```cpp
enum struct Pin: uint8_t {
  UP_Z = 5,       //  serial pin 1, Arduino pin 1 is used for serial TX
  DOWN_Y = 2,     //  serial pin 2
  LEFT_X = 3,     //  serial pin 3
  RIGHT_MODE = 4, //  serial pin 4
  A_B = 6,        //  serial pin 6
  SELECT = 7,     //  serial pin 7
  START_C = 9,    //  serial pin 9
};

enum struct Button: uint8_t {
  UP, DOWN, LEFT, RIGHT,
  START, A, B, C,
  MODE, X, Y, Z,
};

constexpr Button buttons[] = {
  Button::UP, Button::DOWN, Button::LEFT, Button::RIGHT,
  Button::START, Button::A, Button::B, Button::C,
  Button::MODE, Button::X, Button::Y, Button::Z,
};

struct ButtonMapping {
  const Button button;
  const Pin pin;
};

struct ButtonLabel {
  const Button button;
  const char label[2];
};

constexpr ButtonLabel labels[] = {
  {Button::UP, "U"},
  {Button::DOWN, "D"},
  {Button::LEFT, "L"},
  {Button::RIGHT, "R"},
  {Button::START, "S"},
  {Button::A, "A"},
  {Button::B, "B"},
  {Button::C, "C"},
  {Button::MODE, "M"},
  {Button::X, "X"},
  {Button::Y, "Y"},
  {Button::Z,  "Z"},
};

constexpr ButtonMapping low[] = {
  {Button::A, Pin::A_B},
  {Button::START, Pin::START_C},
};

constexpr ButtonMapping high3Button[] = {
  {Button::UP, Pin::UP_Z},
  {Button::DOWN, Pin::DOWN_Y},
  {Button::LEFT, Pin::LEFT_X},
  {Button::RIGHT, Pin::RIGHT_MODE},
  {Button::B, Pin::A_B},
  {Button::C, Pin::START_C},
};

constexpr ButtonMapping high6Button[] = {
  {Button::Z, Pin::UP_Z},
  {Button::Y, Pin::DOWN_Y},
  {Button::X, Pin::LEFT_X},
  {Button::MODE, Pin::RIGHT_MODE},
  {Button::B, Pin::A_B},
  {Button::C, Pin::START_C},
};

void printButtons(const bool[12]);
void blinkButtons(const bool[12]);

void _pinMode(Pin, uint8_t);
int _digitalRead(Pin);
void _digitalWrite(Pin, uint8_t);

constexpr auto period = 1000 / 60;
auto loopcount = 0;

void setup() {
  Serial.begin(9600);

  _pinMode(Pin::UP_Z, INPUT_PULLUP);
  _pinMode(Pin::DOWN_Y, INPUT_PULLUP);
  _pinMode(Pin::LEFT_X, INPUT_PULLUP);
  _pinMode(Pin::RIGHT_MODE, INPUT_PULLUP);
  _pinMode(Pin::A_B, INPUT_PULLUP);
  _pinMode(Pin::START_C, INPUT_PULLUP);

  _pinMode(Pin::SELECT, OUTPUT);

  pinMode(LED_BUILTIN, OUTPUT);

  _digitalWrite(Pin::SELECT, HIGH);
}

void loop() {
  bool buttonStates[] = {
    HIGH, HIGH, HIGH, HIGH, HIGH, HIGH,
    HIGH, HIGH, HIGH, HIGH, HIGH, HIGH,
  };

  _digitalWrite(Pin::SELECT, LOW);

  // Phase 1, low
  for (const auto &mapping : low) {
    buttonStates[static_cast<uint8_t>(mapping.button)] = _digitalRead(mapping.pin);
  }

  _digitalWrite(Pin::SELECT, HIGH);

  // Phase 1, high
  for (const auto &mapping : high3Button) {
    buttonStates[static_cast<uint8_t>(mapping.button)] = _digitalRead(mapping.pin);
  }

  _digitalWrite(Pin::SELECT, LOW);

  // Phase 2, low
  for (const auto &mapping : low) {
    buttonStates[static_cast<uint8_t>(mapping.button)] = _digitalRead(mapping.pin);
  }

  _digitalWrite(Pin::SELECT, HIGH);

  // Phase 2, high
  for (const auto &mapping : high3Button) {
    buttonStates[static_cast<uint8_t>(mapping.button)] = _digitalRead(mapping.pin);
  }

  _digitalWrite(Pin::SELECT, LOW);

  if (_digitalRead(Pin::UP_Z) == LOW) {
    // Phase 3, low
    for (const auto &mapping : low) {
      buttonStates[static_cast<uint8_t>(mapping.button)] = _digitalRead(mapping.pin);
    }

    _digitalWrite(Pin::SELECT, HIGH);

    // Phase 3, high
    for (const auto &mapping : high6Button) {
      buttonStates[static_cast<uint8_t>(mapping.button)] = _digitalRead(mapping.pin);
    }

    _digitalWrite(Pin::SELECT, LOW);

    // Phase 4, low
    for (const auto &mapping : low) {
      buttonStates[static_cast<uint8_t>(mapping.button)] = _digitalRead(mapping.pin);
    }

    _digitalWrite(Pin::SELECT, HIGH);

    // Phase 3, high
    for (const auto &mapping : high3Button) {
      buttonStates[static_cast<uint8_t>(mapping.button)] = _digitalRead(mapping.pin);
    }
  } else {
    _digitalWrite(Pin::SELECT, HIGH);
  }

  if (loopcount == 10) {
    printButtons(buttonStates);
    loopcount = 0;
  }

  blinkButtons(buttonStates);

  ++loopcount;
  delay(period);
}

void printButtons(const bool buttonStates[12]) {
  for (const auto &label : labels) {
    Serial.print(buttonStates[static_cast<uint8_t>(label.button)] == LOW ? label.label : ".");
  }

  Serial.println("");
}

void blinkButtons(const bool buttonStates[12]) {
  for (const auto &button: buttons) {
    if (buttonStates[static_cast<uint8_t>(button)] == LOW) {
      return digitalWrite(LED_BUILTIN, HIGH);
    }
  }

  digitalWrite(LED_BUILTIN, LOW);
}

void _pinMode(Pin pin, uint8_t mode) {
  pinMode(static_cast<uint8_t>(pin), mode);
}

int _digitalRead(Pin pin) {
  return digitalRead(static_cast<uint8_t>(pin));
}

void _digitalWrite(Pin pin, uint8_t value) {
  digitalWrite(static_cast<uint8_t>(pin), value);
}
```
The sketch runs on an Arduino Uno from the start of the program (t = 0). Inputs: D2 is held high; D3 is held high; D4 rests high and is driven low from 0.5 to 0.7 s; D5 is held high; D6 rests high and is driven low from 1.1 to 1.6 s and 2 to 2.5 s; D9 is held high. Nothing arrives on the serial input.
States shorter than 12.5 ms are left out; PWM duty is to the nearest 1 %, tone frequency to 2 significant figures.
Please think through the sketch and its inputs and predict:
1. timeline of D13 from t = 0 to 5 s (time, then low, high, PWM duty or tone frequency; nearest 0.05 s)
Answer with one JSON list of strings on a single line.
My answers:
["0 s low; 0.5 s high; 0.7 s low; 1.1 s high; 1.6 s low; 2 s high; 2.5 s low"]
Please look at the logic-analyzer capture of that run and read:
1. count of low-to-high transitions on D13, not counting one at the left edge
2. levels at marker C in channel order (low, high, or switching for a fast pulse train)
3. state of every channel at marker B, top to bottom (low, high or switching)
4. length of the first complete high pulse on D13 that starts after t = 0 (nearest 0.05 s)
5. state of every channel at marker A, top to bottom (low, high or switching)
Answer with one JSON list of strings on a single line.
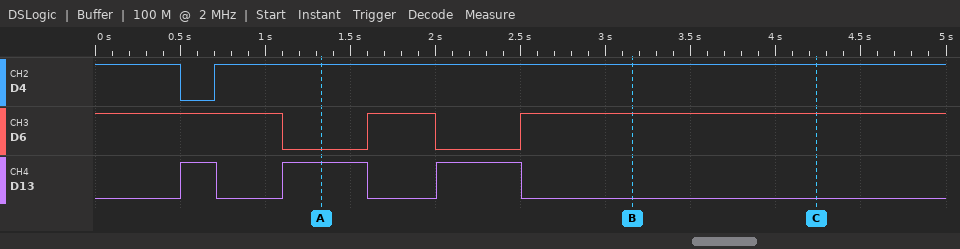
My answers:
["3", "D4 high, D6 high, D13 low", "D4 high, D6 high, D13 low", "0.20 s", "D4 high, D6 low, D13 high"]
